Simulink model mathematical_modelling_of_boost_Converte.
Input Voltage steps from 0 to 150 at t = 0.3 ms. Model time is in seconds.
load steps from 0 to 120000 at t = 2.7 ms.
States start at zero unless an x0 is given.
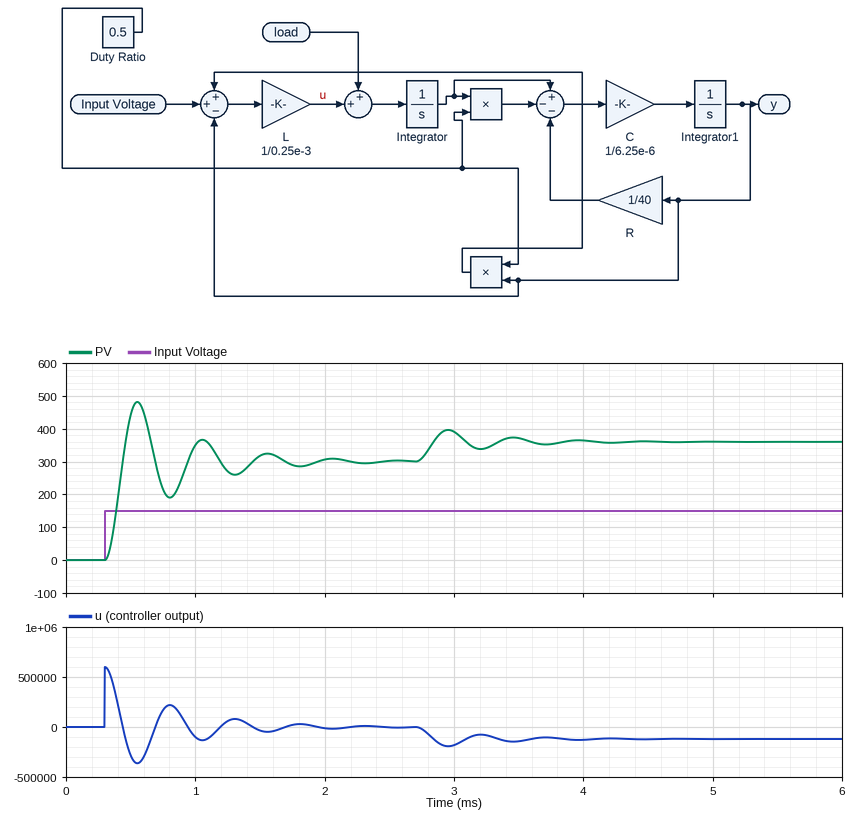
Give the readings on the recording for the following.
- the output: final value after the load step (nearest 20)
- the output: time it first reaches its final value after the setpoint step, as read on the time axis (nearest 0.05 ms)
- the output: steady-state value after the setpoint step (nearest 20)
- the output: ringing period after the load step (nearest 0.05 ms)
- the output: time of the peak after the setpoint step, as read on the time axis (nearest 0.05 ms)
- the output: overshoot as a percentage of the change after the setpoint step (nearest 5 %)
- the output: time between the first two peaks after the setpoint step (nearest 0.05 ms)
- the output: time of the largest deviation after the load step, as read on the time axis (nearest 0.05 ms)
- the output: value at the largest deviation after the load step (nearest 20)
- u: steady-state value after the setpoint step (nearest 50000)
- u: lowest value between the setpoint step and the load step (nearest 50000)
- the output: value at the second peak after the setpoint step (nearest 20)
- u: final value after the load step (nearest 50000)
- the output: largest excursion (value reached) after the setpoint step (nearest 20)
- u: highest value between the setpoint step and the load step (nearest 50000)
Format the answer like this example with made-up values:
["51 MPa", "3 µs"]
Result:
["360", "0.45 ms", "300", "0.50 ms", "0.55 ms", "60 %", "0.50 ms", "2.95 ms", "400", "0", "-350000", "360", "-100000", "480", "600000"]
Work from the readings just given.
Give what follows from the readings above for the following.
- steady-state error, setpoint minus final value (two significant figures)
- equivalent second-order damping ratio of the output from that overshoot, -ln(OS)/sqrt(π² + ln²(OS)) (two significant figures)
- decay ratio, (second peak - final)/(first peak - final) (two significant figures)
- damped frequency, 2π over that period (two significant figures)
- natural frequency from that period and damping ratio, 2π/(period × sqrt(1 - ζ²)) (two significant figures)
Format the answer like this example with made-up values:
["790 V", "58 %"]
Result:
["-150", "0.16", "0.33", "13 rad/ms", "13 rad/ms"]
